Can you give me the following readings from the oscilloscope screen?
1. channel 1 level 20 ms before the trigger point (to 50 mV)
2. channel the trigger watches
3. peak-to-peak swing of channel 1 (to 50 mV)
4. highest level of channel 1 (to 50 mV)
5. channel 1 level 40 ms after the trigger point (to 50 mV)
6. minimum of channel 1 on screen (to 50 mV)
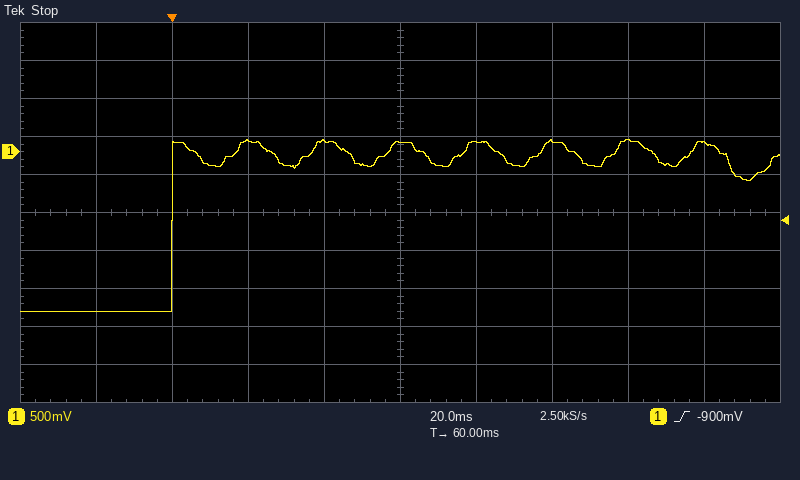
-2.10 V
channel 1
2.25 V
150 mV
150 mV
-2.10 V
